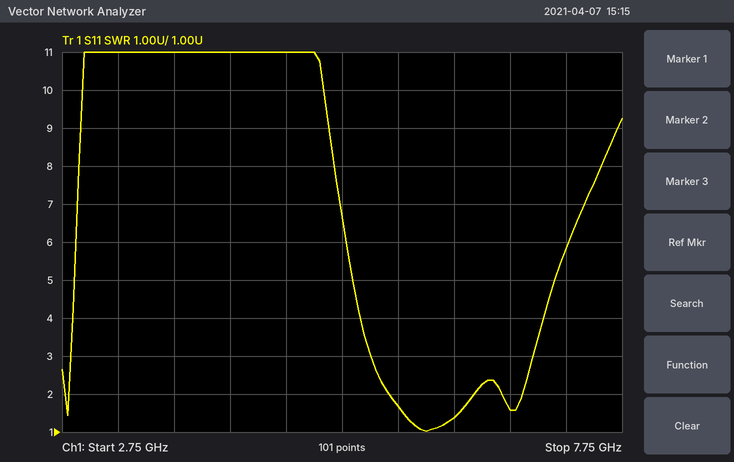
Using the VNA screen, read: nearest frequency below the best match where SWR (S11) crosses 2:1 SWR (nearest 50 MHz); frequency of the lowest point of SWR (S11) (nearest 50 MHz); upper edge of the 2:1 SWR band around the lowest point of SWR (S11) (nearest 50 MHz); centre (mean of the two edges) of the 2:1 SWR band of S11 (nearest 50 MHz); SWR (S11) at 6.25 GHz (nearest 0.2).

5.65 GHz
6.00 GHz
6.45 GHz
6.05 GHz
1.4
